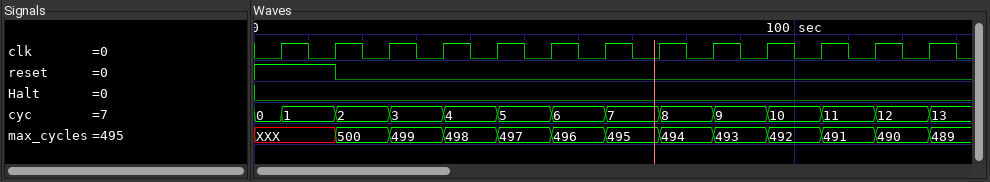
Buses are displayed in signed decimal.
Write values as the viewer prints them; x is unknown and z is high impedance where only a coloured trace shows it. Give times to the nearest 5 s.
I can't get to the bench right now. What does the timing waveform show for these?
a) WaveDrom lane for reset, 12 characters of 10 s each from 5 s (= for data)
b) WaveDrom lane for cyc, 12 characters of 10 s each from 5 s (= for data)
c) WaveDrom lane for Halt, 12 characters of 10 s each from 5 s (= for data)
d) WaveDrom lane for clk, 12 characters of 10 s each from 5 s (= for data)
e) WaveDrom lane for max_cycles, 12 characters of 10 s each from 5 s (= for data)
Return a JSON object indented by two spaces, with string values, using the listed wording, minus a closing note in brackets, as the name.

{
  "WaveDrom lane for reset, 12 characters of 10 s each from 5 s": "{name: 'reset', wave: '10..........'}",
  "WaveDrom lane for cyc, 12 characters of 10 s each from 5 s": "{name: 'cyc', wave: '============', data: '1 2 3 4 5 6 7 8 9 10 11 12'}",
  "WaveDrom lane for Halt, 12 characters of 10 s each from 5 s": "{name: 'Halt', wave: '0...........'}",
  "WaveDrom lane for clk, 12 characters of 10 s each from 5 s": "{name: 'clk', wave: 'p...........'}",
  "WaveDrom lane for max_cycles, 12 characters of 10 s each from 5 s": "{name: 'max_cycles', wave: 'x===========', data: '500 499 498 497 496 495 494 493 492 491 490'}"
}
